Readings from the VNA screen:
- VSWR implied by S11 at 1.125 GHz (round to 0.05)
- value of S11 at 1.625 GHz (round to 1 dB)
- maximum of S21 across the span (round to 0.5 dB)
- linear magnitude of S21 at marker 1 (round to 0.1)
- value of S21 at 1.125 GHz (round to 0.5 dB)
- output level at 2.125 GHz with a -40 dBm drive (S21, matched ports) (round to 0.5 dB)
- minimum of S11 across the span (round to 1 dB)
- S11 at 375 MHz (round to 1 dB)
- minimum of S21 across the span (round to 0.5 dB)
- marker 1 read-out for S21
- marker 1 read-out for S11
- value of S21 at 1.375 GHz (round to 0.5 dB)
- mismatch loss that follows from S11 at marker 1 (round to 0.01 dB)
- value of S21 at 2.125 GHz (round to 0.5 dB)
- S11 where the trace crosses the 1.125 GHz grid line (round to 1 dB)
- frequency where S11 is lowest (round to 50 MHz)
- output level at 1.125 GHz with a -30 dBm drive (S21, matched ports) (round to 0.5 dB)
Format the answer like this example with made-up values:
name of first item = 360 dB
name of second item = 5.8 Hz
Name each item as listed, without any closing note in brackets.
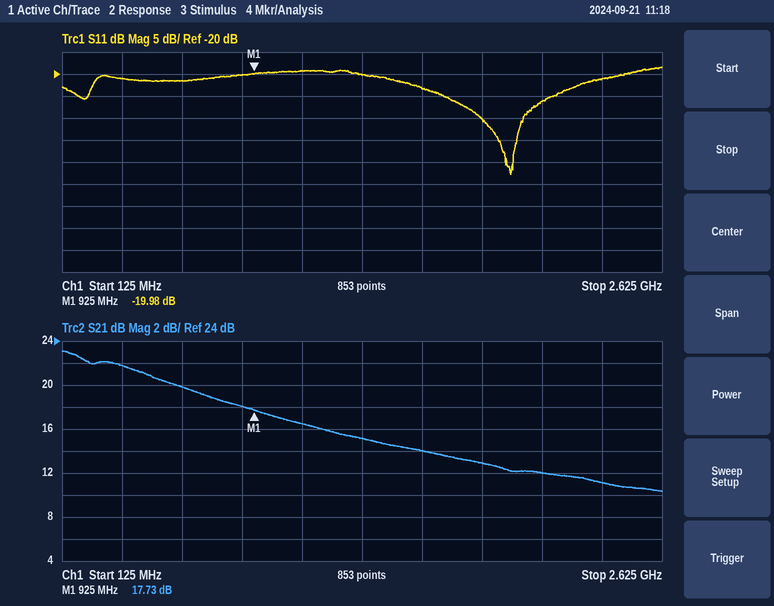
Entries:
VSWR implied by S11 at 1.125 GHz = 1.25
value of S11 at 1.625 GHz = -23 dB
maximum of S21 across the span = 23.0 dB
linear magnitude of S21 at marker 1 = 7.7
value of S21 at 1.125 GHz = 16.5 dB
output level at 2.125 GHz with a -40 dBm drive (S21, matched ports) = -28.0 dBm
minimum of S11 across the span = -43 dB
S11 at 375 MHz = -21 dB
minimum of S21 across the span = 10.5 dB
marker 1 read-out for S21 = 17.73 dB
marker 1 read-out for S11 = -19.98 dB
value of S21 at 1.375 GHz = 15.0 dB
mismatch loss that follows from S11 at marker 1 = 0.04 dB
value of S21 at 2.125 GHz = 12.0 dB
S11 where the trace crosses the 1.125 GHz grid line = -19 dB
frequency where S11 is lowest = 2.00 GHz
output level at 1.125 GHz with a -30 dBm drive (S21, matched ports) = -13.5 dBm
